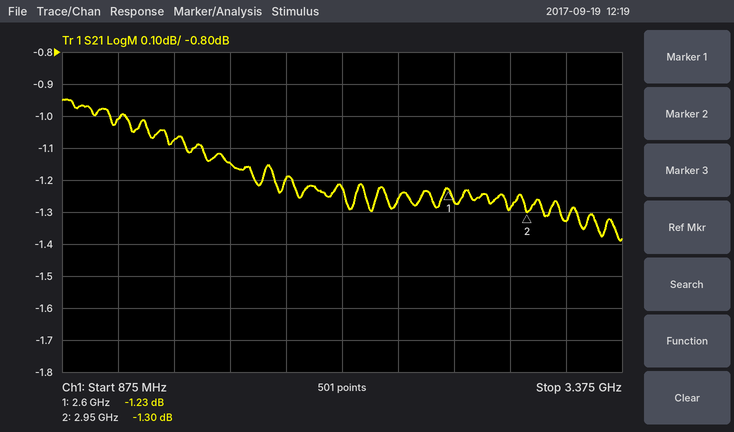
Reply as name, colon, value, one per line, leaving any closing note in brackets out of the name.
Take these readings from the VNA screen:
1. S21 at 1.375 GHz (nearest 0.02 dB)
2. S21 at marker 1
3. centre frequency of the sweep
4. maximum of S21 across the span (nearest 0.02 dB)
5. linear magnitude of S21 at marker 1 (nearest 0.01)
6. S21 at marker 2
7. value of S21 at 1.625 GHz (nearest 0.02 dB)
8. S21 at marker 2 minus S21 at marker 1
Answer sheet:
S21 at 1.375 GHz: -1.08 dB
S21 at marker 1: -1.23 dB
centre frequency of the sweep: 2.125 GHz
maximum of S21 across the span: -0.94 dB
linear magnitude of S21 at marker 1: 0.87
S21 at marker 2: -1.30 dB
value of S21 at 1.625 GHz: -1.14 dB
S21 at marker 2 minus S21 at marker 1: -0.07 dB
